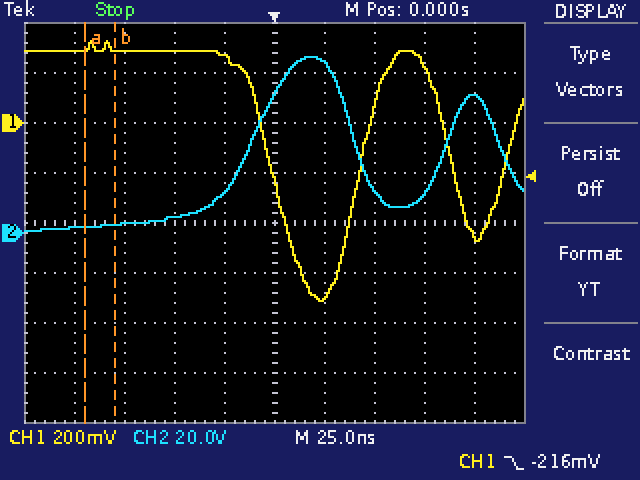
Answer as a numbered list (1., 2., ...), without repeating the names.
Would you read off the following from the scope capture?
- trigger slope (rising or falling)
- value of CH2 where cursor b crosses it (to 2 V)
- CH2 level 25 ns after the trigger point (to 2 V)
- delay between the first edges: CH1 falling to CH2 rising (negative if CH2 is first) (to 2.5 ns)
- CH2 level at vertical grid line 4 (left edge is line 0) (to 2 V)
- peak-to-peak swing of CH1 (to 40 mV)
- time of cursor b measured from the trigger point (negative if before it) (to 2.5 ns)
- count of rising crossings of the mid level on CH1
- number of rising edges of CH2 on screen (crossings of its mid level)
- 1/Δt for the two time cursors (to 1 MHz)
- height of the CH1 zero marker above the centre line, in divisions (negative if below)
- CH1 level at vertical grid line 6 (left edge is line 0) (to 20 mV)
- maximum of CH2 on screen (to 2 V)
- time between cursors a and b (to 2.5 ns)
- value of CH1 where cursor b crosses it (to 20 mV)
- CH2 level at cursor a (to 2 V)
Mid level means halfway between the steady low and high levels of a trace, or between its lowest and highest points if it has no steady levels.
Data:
1. falling
2. 4 V
3. 68 V
4. -10.0 ns
5. 16 V
6. 1.04 V
7. -80.0 ns
8. 2
9. 2
10. 67 MHz
11. +2.0 div
12. -700 mV
13. 70 V
14. 15.0 ns
15. 300 mV
16. 2 V
